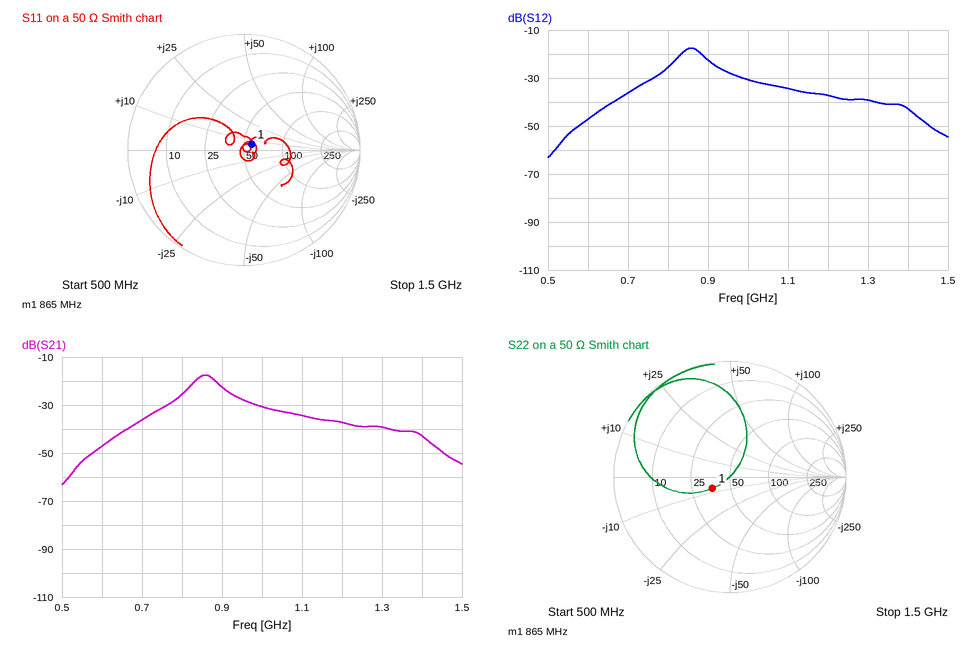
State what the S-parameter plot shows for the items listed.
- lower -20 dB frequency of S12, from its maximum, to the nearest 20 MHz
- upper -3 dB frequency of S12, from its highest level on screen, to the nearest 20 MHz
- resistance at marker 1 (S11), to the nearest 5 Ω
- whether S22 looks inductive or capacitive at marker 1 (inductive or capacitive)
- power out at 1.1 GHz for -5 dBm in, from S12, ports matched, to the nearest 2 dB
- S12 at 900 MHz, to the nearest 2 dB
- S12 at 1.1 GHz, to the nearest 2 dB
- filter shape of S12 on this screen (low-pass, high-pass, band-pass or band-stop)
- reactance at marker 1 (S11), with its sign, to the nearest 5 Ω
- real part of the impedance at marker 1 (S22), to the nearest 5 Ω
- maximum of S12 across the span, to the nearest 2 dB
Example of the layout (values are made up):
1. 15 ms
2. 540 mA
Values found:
1. 680 MHz
2. 880 MHz
3. 55 Ω
4. capacitive
5. -40 dBm
6. -22 dB
7. -34 dB
8. band-pass
9. +5 Ω
10. 35 Ω
11. -18 dB
